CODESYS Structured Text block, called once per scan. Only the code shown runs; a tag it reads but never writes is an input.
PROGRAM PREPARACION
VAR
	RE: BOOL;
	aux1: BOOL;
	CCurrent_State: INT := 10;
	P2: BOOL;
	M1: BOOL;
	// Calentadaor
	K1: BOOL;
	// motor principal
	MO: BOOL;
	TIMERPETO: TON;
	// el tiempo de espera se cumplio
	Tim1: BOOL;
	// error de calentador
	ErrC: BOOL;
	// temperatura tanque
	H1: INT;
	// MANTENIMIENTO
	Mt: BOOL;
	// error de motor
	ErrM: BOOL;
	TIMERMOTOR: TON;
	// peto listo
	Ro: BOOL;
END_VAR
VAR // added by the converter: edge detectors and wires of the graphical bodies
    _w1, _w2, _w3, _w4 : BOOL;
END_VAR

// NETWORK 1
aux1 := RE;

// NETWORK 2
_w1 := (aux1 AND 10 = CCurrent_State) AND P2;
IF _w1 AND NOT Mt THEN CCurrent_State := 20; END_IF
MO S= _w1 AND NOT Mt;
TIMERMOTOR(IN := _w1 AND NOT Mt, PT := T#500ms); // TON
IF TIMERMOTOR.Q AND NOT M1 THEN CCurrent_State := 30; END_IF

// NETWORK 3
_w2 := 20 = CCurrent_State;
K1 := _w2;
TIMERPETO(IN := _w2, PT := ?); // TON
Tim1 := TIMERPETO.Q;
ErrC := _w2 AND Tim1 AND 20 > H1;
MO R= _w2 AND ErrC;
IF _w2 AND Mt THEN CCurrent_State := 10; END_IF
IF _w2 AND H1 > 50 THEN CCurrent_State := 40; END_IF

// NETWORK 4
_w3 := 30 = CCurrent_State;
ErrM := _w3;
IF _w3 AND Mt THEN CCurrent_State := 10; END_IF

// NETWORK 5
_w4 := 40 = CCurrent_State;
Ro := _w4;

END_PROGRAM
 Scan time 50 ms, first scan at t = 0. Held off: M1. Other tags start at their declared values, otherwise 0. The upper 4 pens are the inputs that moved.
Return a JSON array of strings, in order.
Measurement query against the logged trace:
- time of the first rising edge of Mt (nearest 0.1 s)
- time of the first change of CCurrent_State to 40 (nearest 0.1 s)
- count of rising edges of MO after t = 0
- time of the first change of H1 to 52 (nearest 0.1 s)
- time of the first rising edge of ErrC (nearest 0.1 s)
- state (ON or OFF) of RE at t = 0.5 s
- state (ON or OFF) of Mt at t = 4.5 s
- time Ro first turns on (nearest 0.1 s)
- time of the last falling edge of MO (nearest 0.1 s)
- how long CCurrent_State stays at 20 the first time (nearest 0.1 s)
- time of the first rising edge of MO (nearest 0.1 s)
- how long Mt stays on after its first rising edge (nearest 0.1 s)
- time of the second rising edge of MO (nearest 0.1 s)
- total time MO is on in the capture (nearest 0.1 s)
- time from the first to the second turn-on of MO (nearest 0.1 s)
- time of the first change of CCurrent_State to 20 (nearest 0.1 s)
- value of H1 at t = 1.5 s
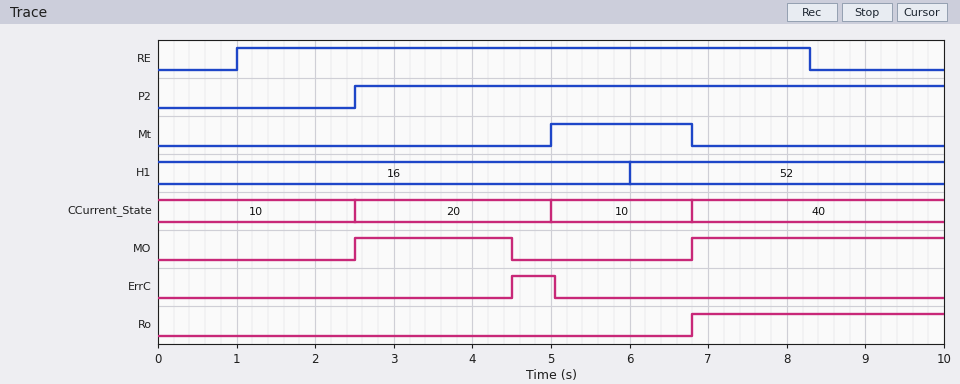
["5.0 s", "6.8 s", "2", "6.0 s", "4.5 s", "OFF", "OFF", "6.8 s", "4.5 s", "2.5 s", "2.5 s", "1.8 s", "6.8 s", "5.2 s", "4.3 s", "2.5 s", "16"]
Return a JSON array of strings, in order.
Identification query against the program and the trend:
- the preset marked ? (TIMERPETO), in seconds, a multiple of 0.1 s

["2.0 s"]
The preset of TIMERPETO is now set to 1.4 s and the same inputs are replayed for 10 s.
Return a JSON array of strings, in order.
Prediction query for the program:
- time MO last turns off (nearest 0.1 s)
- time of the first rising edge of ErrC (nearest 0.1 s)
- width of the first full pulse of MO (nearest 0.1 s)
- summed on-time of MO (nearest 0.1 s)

["3.9 s", "3.9 s", "1.4 s", "4.6 s"]
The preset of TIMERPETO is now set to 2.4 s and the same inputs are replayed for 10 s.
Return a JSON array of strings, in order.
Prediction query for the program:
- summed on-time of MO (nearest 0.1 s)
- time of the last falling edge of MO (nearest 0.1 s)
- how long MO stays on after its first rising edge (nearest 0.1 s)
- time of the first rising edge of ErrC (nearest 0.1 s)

["5.6 s", "4.9 s", "2.4 s", "4.9 s"]
